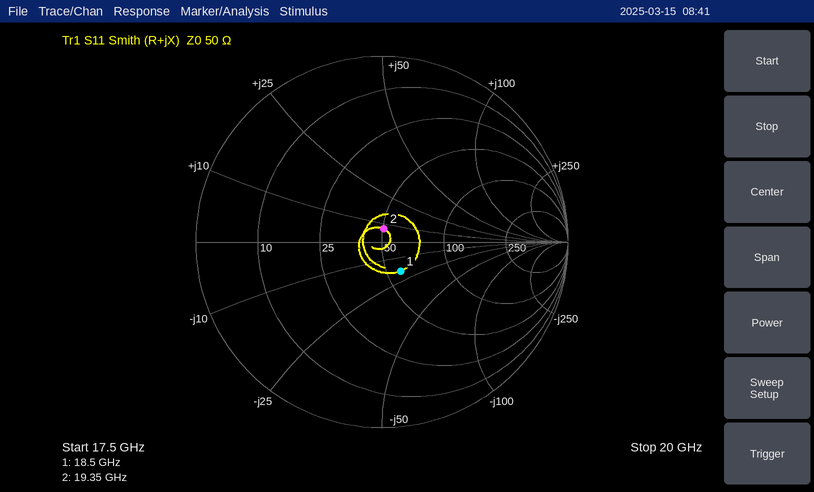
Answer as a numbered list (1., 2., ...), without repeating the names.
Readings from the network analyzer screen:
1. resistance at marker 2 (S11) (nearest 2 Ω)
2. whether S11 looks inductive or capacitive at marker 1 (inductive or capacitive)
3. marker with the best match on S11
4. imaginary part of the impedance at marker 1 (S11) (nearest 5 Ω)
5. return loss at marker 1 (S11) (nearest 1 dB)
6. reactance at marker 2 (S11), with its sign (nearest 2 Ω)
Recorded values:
1. 50 Ω
2. capacitive
3. marker 2
4. -20 Ω
5. 15 dB
6. +8 Ω
